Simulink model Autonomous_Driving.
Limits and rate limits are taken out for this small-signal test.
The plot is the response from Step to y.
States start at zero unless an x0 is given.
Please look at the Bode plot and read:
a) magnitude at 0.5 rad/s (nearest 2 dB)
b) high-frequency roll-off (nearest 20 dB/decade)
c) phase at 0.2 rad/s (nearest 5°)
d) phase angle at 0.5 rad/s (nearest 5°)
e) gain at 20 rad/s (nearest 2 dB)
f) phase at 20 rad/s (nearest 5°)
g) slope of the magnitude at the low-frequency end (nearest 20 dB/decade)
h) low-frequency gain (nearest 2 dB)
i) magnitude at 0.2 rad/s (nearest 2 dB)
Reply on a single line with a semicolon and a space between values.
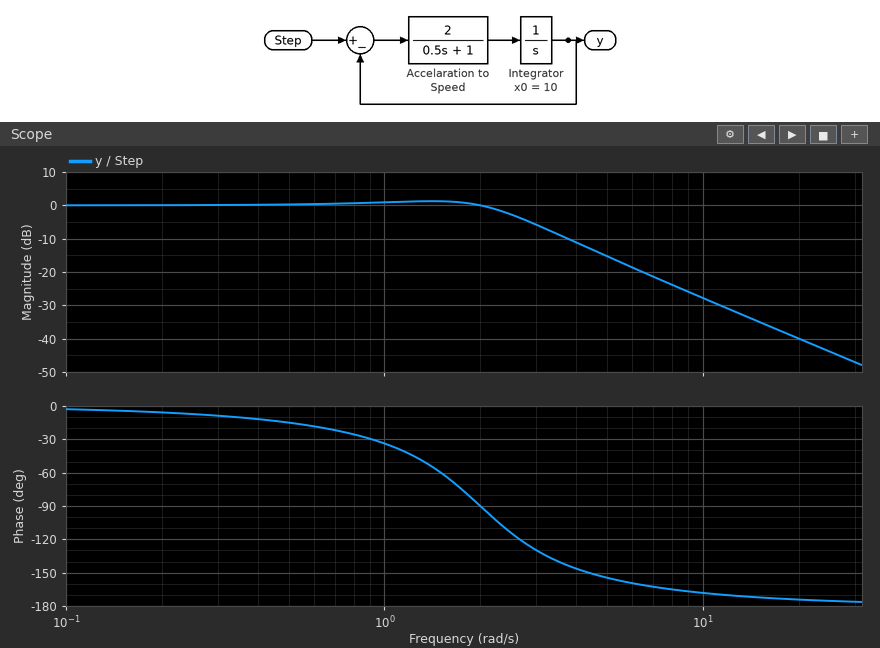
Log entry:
0 dB; -40 dB/decade; -5°; -15°; -40 dB; -175°; 0 dB/decade; 0 dB; 0 dB
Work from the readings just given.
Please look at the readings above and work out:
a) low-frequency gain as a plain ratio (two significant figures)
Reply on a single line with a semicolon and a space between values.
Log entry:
1.0
